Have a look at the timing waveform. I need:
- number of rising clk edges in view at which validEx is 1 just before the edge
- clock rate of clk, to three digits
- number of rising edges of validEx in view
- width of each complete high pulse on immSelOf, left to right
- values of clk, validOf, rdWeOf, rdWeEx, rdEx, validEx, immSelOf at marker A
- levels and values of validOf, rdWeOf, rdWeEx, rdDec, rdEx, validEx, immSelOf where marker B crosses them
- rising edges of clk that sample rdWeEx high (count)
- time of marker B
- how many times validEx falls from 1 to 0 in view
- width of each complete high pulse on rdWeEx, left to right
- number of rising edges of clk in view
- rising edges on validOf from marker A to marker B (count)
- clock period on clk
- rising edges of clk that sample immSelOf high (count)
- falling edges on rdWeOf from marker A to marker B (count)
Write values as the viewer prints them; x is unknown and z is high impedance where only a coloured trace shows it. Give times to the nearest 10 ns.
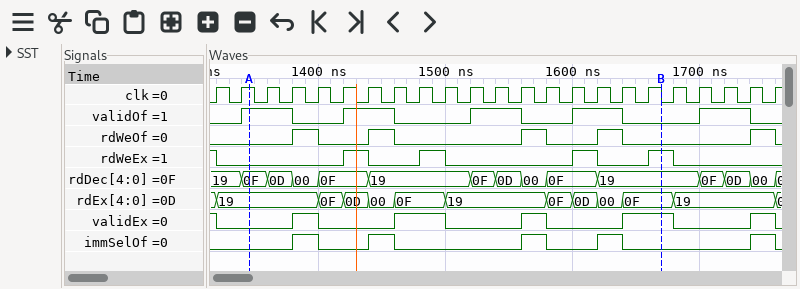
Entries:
8
50.0 MHz
5
20 ns, 20 ns, 20 ns, 20 ns, 20 ns
clk=1, validOf=1, rdWeOf=0, rdWeEx=0, rdEx=19, validEx=0, immSelOf=0
validOf=0, rdWeOf=0, rdWeEx=1, rdDec=19, rdEx=0F, validEx=1, immSelOf=0
5
1670 ns
6
20 ns, 20 ns, 20 ns, 20 ns
23
3
20 ns
5
4
